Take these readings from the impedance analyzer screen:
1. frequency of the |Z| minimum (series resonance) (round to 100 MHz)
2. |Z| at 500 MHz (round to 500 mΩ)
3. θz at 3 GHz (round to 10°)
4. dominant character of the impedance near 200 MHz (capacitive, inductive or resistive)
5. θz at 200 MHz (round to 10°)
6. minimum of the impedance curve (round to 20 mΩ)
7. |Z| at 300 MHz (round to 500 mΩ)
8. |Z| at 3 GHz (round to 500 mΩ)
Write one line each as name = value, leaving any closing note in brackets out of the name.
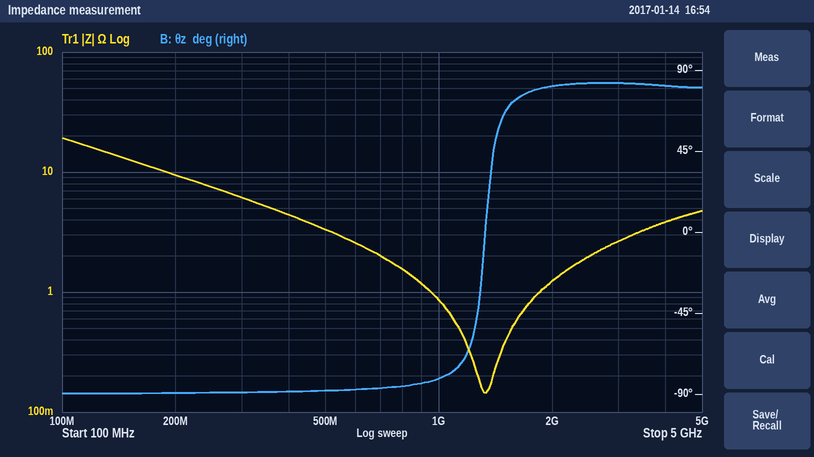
frequency of the |Z| minimum (series resonance) = 1.3 GHz
|Z| at 500 MHz = 3.5 Ω
θz at 3 GHz = 80°
dominant character of the impedance near 200 MHz = capacitive
θz at 200 MHz = -90°
minimum of the impedance curve = 140 mΩ
|Z| at 300 MHz = 6.0 Ω
|Z| at 3 GHz = 2.5 Ω
